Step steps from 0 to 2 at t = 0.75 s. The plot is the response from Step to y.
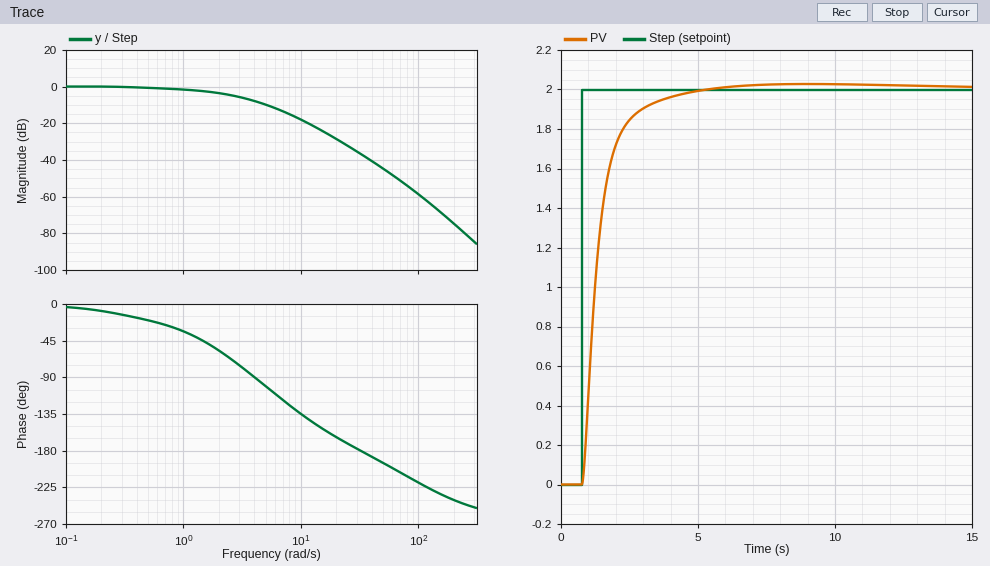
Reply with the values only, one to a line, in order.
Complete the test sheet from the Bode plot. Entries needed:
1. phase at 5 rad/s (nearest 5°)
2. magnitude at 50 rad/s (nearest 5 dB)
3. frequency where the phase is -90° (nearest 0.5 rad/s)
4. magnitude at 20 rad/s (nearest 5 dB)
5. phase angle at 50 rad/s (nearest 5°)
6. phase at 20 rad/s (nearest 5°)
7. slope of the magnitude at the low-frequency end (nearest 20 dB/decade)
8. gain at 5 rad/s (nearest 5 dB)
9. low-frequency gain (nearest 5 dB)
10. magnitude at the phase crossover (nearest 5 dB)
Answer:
-100°
-45 dB
4.0 rad/s
-30 dB
-195°
-165°
0 dB/decade
-10 dB
0 dB
-35 dB
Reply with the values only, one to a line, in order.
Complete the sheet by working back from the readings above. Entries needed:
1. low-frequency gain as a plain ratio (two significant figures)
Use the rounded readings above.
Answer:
1.0
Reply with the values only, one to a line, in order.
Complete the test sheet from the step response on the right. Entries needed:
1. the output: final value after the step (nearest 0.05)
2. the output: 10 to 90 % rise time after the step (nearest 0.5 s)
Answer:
2.00
1.5 s
